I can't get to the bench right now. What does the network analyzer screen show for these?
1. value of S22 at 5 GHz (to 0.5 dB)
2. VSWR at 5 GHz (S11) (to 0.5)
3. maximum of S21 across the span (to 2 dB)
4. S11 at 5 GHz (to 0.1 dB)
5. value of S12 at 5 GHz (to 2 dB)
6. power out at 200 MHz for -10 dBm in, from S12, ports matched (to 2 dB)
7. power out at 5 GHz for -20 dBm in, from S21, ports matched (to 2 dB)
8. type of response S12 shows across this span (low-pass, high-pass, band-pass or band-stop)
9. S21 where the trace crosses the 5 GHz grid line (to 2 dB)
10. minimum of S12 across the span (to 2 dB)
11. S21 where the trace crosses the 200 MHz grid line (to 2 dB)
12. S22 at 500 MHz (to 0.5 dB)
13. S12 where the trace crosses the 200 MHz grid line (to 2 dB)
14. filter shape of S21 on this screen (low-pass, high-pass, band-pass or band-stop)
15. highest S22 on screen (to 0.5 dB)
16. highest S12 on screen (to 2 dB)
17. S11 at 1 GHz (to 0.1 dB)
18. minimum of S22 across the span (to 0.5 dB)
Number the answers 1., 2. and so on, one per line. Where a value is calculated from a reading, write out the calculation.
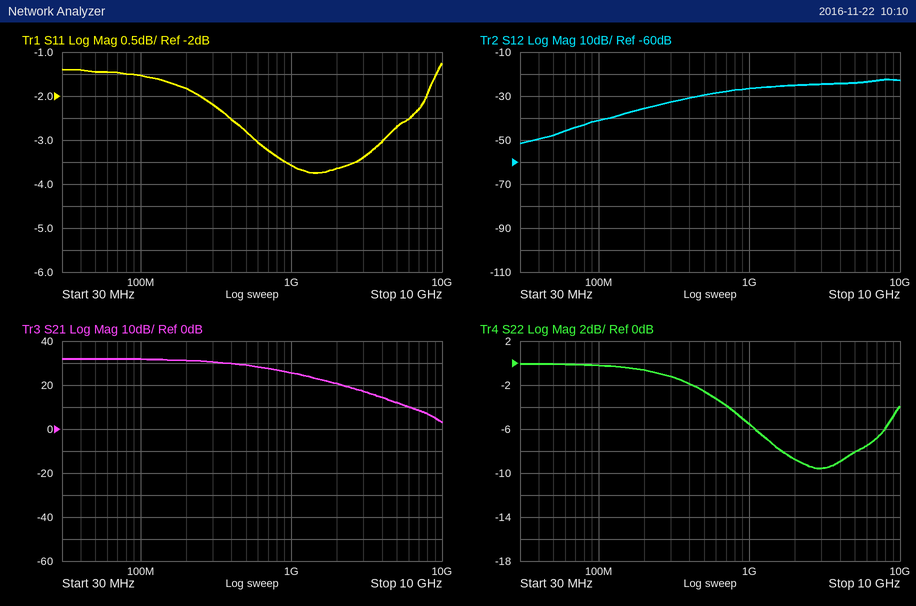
1. -8.0 dB
2. |Γ| = 10^(-2.7/20) = 0.7328; VSWR = (1 + 0.7328)/(1 − 0.7328) ≈ 6.5
3. 32 dB
4. -2.7 dB
5. -24 dB
6. -10 dBm + (-36 dB) = -46 dBm
7. -20 dBm + (12 dB) = -8 dBm
8. high-pass
9. 12 dB
10. -52 dB
11. 32 dB
12. -2.5 dB
13. -36 dB
14. low-pass
15. 0.0 dB
16. -22 dB
17. -3.6 dB
18. -9.5 dB
